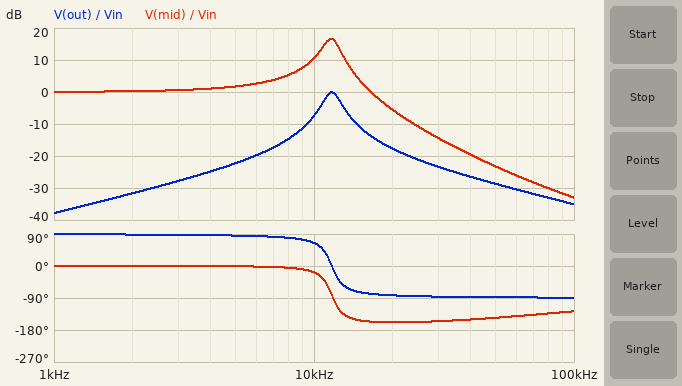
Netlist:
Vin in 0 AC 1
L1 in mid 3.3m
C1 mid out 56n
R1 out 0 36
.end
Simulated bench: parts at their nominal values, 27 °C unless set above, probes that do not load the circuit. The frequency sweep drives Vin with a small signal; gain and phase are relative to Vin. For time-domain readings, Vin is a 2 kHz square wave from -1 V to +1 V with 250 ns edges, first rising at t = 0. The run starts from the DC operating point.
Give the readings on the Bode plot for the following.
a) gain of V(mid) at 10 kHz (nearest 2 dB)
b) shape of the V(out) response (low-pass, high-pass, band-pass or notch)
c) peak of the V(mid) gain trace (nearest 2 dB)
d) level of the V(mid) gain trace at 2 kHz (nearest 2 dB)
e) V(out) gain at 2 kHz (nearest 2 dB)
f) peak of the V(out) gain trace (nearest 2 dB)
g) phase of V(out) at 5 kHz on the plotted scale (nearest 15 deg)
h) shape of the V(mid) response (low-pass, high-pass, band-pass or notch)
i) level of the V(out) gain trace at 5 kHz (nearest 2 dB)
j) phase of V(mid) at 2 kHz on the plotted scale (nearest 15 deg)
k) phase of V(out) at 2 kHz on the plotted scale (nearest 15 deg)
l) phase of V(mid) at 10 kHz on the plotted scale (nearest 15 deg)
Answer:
10 dB
band-pass
16 dB
0 dB
-32 dB
0 dB
90 deg
low-pass
-22 dB
0 deg
90 deg
-15 deg
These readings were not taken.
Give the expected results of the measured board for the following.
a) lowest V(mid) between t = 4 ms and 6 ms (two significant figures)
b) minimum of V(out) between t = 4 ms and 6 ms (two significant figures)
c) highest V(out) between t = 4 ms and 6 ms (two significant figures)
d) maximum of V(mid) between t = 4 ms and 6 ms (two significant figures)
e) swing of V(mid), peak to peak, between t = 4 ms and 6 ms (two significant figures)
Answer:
-2.3 V
-220 mV
220 mV
2.3 V
4.6 V
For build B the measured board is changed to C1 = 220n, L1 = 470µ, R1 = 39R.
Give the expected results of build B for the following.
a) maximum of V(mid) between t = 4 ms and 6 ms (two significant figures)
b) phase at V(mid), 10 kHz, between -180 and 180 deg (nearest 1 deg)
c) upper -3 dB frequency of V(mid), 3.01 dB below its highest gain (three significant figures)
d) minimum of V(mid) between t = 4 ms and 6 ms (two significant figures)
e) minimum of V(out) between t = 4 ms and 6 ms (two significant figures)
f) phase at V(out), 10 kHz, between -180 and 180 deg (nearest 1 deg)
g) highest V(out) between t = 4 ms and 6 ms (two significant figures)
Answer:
1.7 V
-14 deg
20.5 kHz
-1.7 V
-1.0 V
48 deg
1.0 V
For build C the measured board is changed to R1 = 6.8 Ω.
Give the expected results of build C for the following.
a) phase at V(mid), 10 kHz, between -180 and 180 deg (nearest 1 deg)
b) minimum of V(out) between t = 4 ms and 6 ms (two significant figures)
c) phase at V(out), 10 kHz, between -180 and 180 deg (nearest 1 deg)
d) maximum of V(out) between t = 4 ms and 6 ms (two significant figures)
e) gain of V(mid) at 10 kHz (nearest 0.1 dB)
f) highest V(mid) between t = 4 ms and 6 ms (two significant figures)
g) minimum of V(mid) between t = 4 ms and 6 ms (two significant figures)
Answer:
-4 deg
-32 mV
85 deg
32 mV
11.3 dB
2.1 V
-2.1 V
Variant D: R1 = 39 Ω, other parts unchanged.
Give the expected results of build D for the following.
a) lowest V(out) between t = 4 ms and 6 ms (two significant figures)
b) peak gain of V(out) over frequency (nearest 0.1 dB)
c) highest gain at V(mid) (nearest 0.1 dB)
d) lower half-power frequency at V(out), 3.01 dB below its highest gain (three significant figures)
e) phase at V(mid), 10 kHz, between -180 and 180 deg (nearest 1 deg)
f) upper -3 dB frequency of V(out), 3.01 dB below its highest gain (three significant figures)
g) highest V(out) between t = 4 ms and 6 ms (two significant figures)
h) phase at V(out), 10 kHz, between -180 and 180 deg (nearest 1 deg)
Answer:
-240 mV
0 dB
16.0 dB
10.8 kHz
-19 deg
12.7 kHz
240 mV
63 deg
